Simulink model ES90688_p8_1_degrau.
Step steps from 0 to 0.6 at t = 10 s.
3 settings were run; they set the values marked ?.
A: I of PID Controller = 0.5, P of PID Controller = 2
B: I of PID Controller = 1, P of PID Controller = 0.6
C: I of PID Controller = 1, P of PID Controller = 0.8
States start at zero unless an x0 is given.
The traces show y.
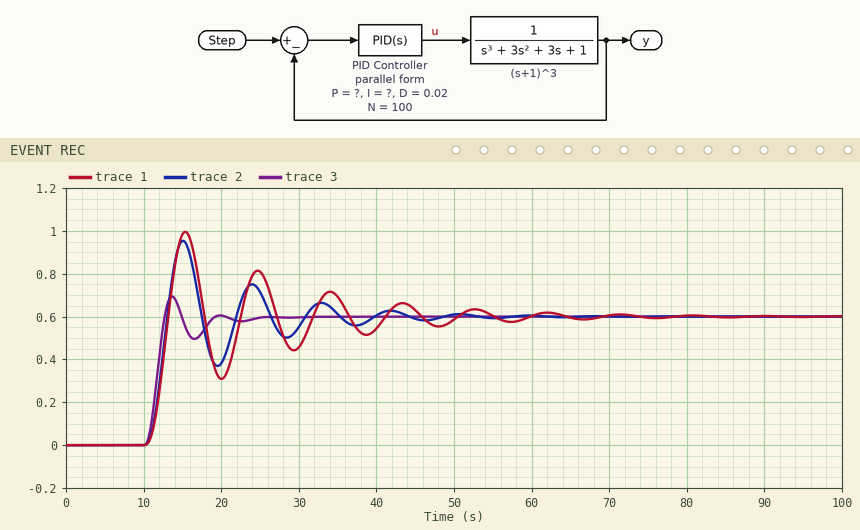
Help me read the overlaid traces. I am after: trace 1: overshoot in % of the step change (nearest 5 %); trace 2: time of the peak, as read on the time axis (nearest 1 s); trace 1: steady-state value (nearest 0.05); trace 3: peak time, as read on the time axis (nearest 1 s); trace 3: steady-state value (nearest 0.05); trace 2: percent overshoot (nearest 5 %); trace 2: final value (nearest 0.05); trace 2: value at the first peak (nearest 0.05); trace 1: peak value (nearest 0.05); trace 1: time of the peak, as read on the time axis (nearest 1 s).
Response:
65 %
15 s
0.60
14 s
0.60
60 %
0.60
0.95
1.00
15 s
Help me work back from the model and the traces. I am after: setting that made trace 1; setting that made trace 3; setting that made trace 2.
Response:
B
A
C
